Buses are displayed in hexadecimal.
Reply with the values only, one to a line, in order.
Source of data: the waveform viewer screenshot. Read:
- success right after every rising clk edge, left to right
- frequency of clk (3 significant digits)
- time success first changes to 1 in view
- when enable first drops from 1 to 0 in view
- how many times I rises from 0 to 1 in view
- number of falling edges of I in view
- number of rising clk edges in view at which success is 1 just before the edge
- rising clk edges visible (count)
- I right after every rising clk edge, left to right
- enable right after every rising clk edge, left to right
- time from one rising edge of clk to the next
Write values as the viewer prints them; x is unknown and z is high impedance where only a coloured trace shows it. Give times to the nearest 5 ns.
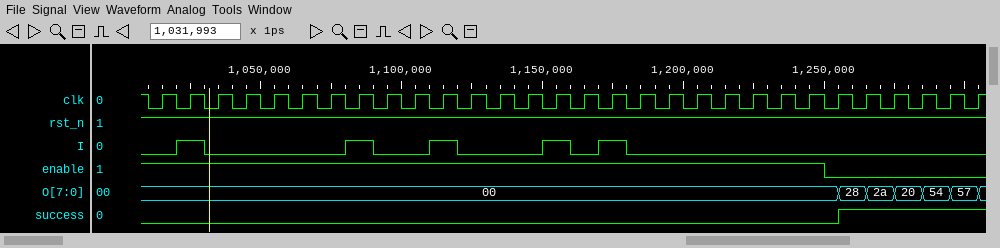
0 0 0 0 0 0 0 0 0 0 0 0 0 0 0 0 0 0 0 0 0 0 0 0 1 1 1 1 1 1
100 MHz
1255 ns
1250 ns
5
5
5
30
0 1 0 0 0 0 0 1 0 0 1 0 0 0 1 0 1 0 0 0 0 0 0 0 0 0 0 0 0 0
1 1 1 1 1 1 1 1 1 1 1 1 1 1 1 1 1 1 1 1 1 1 1 1 0 0 0 0 0 0
10 ns
